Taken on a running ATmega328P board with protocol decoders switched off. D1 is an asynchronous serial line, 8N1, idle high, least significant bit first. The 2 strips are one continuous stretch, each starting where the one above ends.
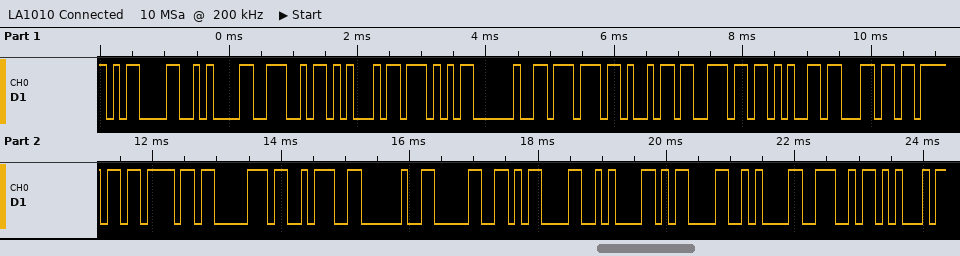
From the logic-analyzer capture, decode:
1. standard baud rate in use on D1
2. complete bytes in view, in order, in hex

9600 baud
0D 0A 4E 45 57 20 77 69 6E 65 6C 6F 6F 70 3A 20 30 0D 0A 0D 0A 4E 45
